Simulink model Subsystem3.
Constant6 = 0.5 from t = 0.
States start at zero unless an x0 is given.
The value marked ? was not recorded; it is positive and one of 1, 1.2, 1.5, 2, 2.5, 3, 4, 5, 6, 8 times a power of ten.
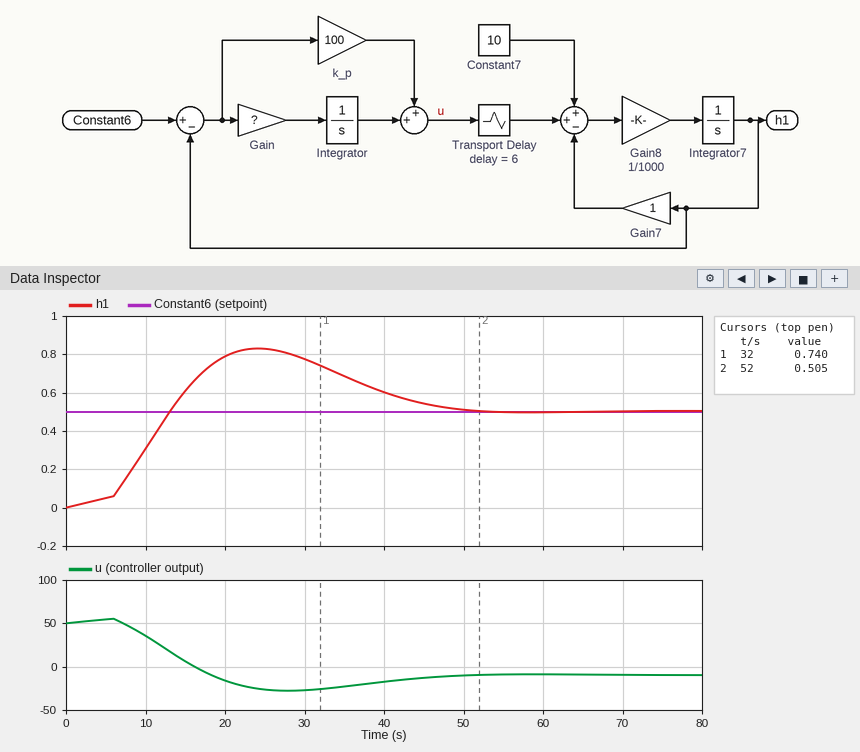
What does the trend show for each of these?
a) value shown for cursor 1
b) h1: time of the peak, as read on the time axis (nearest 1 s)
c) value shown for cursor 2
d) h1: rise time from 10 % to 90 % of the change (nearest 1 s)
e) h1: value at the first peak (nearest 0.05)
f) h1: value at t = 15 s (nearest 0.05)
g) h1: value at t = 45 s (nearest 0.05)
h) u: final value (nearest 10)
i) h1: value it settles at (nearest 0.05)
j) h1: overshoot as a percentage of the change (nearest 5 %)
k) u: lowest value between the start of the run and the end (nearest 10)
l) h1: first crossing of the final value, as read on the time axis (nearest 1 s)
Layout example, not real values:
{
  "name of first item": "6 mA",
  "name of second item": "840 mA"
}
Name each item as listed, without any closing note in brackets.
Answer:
{
  "value shown for cursor 1": "0.740",
  "h1: time of the peak, as read on the time axis": "24 s",
  "value shown for cursor 2": "0.505",
  "h1: rise time from 10 % to 90 % of the change": "7 s",
  "h1: value at the first peak": "0.85",
  "h1: value at t = 15 s": "0.60",
  "h1: value at t = 45 s": "0.55",
  "u: final value": "-10",
  "h1: value it settles at": "0.50",
  "h1: overshoot as a percentage of the change": "65 %",
  "u: lowest value between the start of the run and the end": "-30",
  "h1: first crossing of the final value, as read on the time axis": "13 s"
}
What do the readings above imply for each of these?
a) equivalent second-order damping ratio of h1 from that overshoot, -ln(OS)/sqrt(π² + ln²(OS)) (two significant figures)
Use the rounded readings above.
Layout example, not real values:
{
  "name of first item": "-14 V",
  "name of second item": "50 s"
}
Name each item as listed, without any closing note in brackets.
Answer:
{
  "equivalent second-order damping ratio of h1 from that overshoot, -ln(OS)/sqrt(π² + ln²(OS))": "0.14"
}
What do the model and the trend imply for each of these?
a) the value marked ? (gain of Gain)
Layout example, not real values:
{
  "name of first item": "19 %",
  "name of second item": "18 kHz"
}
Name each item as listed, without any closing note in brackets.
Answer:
{
  "the value marked ?": "4"
}
